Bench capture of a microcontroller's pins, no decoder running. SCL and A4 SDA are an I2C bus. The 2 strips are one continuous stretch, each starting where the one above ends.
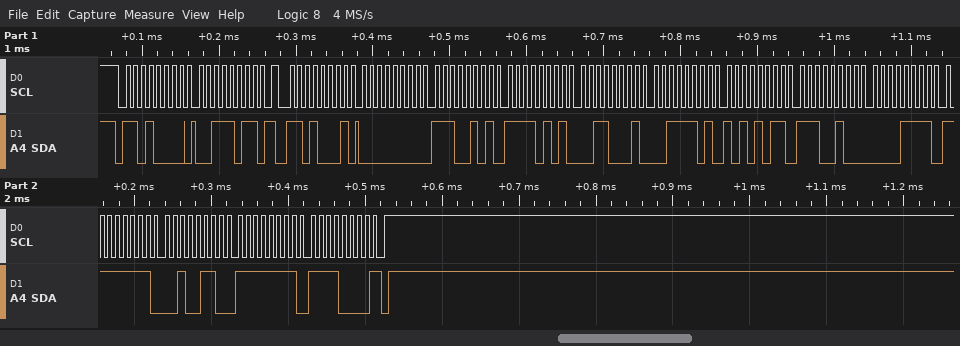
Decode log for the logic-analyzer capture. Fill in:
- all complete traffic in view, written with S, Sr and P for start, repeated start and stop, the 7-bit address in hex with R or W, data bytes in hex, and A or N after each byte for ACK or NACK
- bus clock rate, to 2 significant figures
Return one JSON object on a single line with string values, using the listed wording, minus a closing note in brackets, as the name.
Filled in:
{"all complete traffic in view, written with S, Sr and P for start, repeated start and stop, the 7-bit address in hex with R or W, data bytes in hex, and A or N after each byte for ACK or NACK": "S 68W A 3B A Sr 68R A 00 A E5 A F5 A 31 A 3D A AB A E4 A 0F A FF A 26 A FF A F0 N P", "bus clock rate, to 2 significant figures": "100 kHz"}
